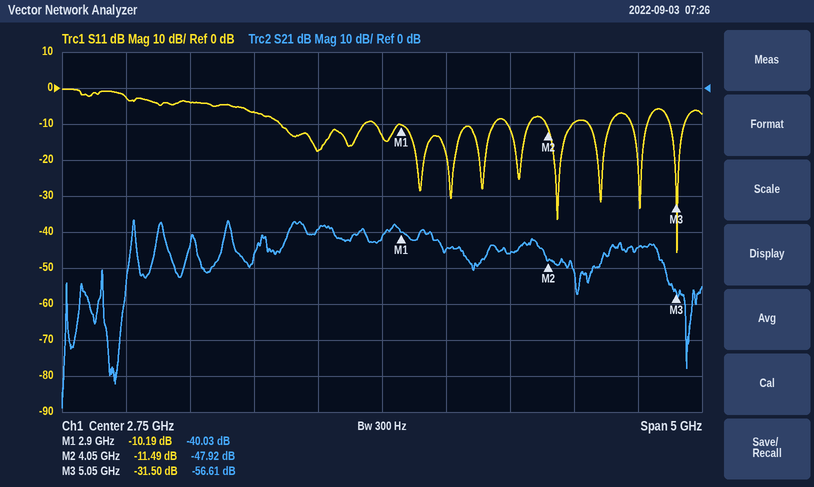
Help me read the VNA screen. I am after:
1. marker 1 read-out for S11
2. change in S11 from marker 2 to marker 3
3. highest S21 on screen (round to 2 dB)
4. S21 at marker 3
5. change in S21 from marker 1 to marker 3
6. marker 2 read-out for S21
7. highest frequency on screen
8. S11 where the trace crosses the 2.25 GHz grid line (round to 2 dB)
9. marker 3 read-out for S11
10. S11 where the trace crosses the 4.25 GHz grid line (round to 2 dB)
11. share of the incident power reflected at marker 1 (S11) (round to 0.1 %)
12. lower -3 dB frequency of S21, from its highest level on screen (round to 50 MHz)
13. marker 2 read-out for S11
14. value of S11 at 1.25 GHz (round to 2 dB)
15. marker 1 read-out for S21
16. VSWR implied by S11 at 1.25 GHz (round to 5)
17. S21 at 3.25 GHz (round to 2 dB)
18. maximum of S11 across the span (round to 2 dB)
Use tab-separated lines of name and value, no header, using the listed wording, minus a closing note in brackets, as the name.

marker 1 read-out for S11	-10.19 dB
change in S11 from marker 2 to marker 3	-20.01 dB
highest S21 on screen	-36 dB
S21 at marker 3	-56.61 dB
change in S21 from marker 1 to marker 3	-16.58 dB
marker 2 read-out for S21	-47.92 dB
highest frequency on screen	5.25 GHz
S11 where the trace crosses the 2.25 GHz grid line	-18 dB
marker 3 read-out for S11	-31.50 dB
S11 where the trace crosses the 4.25 GHz grid line	-10 dB
share of the incident power reflected at marker 1 (S11)	9.6 %
lower -3 dB frequency of S21, from its highest level on screen	800 MHz
marker 2 read-out for S11	-11.49 dB
value of S11 at 1.25 GHz	-4 dB
marker 1 read-out for S21	-40.03 dB
VSWR implied by S11 at 1.25 GHz	5
S21 at 3.25 GHz	-44 dB
maximum of S11 across the span	0 dB
